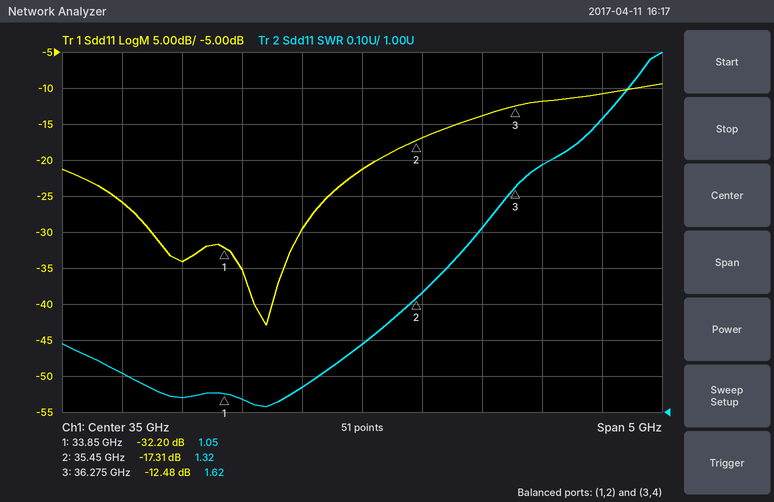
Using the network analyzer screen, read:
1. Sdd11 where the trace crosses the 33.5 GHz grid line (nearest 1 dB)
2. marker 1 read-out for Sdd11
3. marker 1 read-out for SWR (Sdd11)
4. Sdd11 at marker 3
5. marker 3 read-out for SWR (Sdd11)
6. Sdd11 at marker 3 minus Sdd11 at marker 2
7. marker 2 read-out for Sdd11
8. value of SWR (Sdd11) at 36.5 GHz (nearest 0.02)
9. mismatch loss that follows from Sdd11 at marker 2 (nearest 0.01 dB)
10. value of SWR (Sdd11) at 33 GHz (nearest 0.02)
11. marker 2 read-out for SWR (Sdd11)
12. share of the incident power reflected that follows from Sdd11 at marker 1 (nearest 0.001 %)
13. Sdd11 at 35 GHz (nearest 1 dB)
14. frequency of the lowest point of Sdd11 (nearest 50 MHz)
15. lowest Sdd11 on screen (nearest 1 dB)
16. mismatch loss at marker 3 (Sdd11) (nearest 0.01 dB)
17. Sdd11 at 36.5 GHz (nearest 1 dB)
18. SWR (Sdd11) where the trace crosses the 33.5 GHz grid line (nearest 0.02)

-34 dB
-32.20 dB
1.05
-12.48 dB
1.62
4.83 dB
-17.31 dB
1.68
0.08 dB
1.10
1.32
0.060 %
-21 dB
34.20 GHz
-43 dB
0.25 dB
-12 dB
1.04
